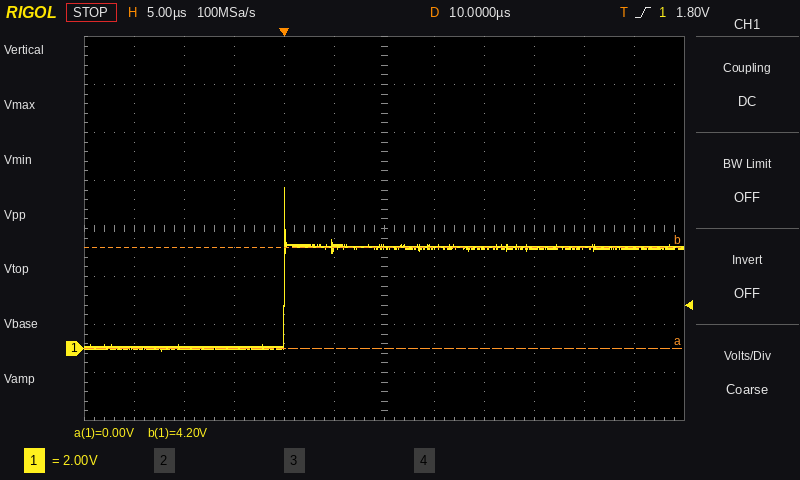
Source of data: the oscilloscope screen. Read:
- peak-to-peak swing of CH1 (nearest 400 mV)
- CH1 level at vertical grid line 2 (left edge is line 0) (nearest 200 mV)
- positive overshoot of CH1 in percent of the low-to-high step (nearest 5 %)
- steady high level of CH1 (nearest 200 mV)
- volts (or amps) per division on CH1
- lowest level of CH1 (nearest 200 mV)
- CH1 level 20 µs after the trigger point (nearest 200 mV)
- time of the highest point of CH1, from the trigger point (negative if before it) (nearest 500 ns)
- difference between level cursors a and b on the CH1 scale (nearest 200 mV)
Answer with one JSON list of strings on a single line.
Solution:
["6.8 V", "0.0 V", "60 %", "4.2 V", "2 V", "0.0 V", "4.2 V", "0.0 µs", "4.2 V"]
